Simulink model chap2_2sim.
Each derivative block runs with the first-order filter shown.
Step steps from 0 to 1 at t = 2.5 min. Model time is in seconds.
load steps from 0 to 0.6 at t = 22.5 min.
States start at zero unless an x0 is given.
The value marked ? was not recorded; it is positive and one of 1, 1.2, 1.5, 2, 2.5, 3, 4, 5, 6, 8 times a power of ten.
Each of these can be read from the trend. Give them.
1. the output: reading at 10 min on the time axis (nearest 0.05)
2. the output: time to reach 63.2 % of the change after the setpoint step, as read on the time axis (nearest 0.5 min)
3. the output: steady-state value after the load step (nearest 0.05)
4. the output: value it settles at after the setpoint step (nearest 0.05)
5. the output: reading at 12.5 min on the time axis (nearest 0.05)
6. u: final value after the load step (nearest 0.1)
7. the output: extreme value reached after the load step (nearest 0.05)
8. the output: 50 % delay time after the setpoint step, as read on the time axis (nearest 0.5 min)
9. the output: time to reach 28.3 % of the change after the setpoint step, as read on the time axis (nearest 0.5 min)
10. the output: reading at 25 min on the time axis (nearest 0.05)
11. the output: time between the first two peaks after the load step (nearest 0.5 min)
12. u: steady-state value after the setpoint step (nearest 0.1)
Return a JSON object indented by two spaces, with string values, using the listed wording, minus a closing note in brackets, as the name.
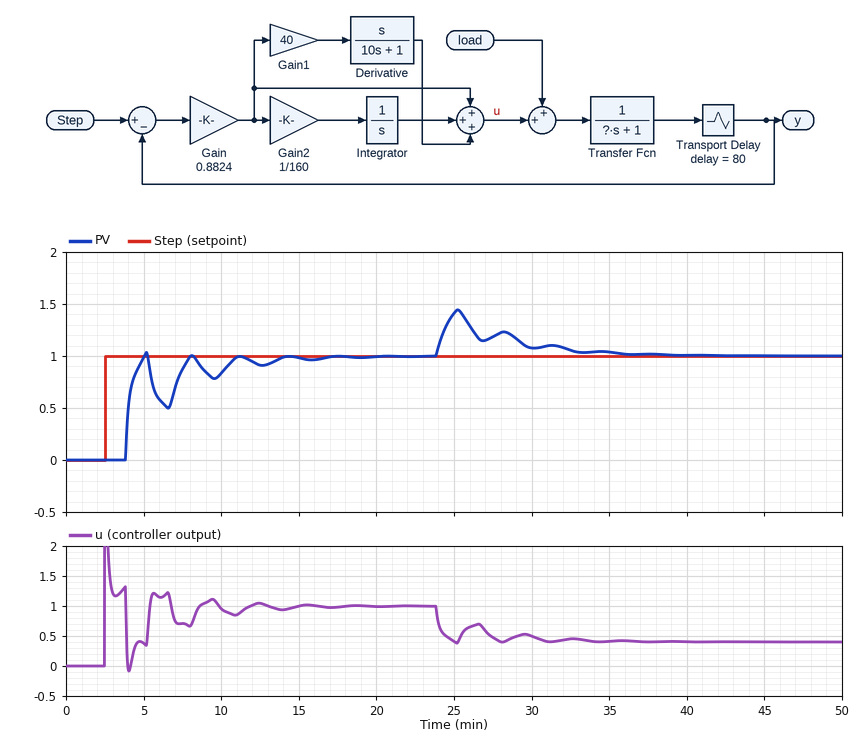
{
  "the output: reading at 10 min on the time axis": "0.85",
  "the output: time to reach 63.2 % of the change after the setpoint step, as read on the time axis": "4.0 min",
  "the output: steady-state value after the load step": "1.00",
  "the output: value it settles at after the setpoint step": "1.00",
  "the output: reading at 12.5 min on the time axis": "0.90",
  "u: final value after the load step": "0.4",
  "the output: extreme value reached after the load step": "1.45",
  "the output: 50 % delay time after the setpoint step, as read on the time axis": "4.0 min",
  "the output: time to reach 28.3 % of the change after the setpoint step, as read on the time axis": "4.0 min",
  "the output: reading at 25 min on the time axis": "1.40",
  "the output: time between the first two peaks after the load step": "3.0 min",
  "u: steady-state value after the setpoint step": "1.0"
}
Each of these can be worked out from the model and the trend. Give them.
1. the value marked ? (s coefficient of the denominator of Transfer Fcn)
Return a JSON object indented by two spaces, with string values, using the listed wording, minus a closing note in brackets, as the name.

{
  "the value marked ?": "60"
}
